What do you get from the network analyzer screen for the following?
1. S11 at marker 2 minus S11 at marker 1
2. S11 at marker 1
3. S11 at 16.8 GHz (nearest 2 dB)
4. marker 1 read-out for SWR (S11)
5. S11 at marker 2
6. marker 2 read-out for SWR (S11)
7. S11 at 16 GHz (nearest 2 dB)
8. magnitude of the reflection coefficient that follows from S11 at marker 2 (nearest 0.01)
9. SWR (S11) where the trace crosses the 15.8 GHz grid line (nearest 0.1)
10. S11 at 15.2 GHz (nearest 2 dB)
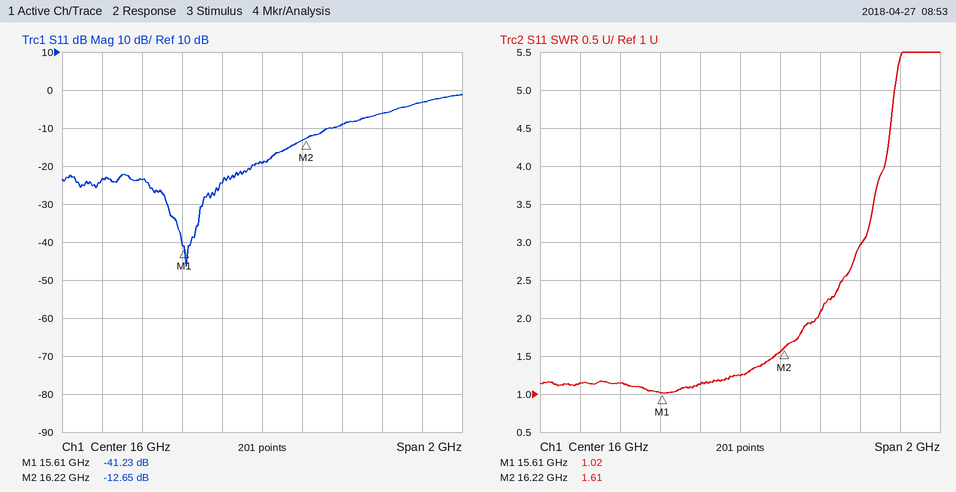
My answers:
28.58 dB
-41.23 dB
-4 dB
1.02
-12.65 dB
1.61
-20 dB
0.23
1.1
-24 dB
